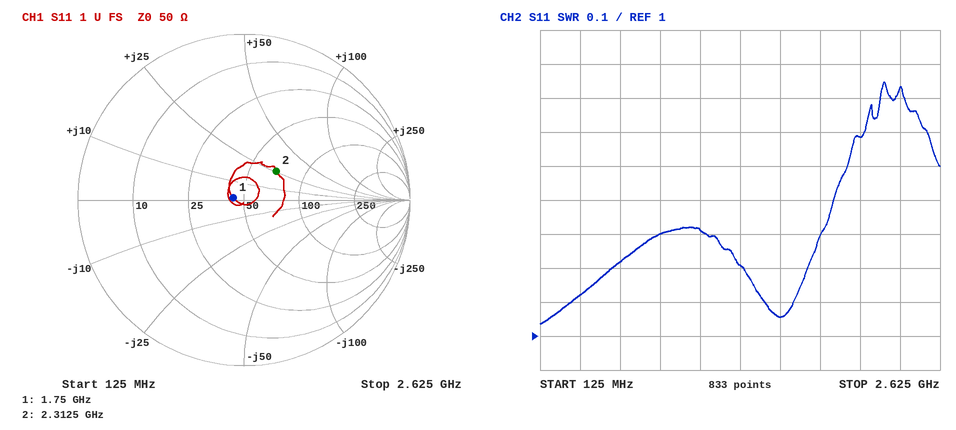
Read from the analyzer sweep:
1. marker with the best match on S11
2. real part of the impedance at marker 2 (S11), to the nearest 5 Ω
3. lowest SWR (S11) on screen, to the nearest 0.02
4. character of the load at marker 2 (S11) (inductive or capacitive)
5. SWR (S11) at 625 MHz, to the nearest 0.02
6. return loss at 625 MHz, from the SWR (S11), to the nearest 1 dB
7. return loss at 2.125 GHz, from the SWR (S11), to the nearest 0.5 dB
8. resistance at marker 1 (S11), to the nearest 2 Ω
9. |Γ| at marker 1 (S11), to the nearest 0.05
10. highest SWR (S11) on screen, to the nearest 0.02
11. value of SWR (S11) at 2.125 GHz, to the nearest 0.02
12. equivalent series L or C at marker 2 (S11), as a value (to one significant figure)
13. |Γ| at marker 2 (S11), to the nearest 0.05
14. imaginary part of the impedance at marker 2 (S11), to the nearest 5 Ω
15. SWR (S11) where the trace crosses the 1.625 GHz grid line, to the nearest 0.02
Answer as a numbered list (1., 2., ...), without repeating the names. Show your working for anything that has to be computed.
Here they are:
1. marker 1
2. 70 Ω
3. 1.04
4. inductive
5. 1.22
6. −20 log10((1.22 − 1)/(1.22 + 1)) ≈ 20 dB
7. −20 log10((1.58 − 1)/(1.58 + 1)) ≈ 13.0 dB
8. 44 Ω
9. 0.05
10. 1.74
11. 1.58
12. L = 25 Ω/(2π × 2.3125 GHz) ≈ 2 nH
13. 0.25
14. +25 Ω
15. 1.06
